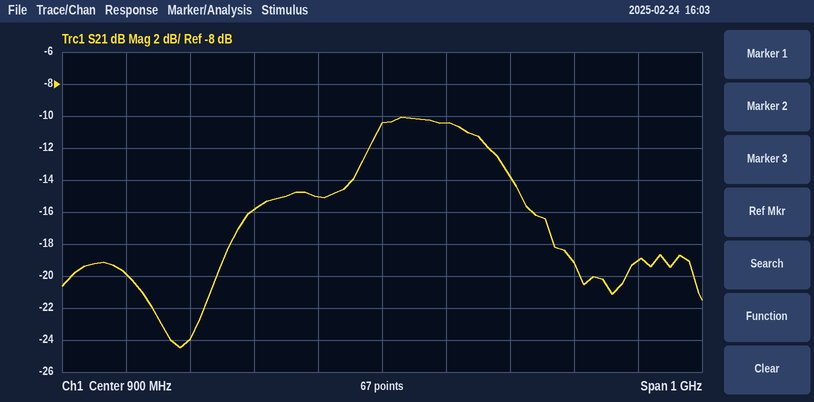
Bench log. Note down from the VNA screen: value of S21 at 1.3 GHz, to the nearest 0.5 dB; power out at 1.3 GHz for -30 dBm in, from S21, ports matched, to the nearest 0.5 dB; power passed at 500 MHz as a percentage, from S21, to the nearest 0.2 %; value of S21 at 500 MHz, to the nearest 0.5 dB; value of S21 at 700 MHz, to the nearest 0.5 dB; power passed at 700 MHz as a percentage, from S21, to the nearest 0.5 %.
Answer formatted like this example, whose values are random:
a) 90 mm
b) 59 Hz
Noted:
a) -19.0 dB
b) -49.0 dBm
c) 1.0 %
d) -20.0 dB
e) -16.0 dB
f) 2.5 %
